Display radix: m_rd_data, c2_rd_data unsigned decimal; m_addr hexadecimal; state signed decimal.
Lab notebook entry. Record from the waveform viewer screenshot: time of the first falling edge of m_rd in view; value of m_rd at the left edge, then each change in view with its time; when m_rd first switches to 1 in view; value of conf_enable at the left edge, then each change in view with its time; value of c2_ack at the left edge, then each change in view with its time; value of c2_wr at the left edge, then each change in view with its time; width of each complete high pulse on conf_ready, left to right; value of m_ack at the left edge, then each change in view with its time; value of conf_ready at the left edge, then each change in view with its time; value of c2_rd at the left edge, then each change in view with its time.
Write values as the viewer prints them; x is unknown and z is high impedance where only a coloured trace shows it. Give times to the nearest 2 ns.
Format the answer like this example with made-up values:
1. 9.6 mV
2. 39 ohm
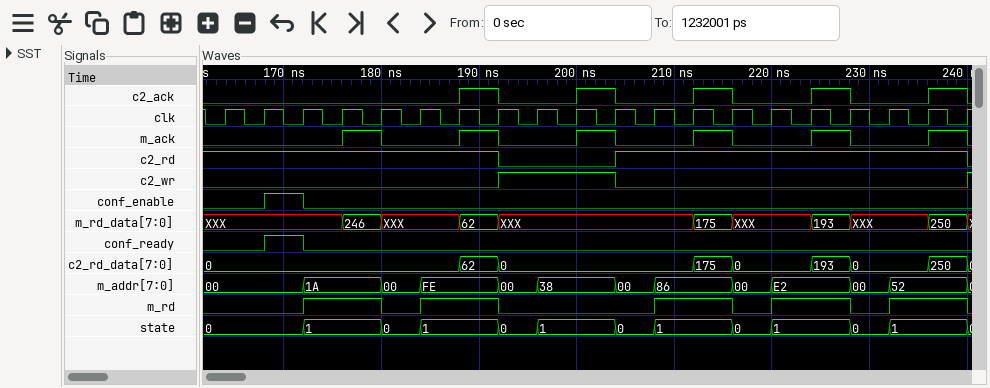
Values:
1. 180 ns
2. 0, 1 at 172 ns, 0 at 180 ns, 1 at 184 ns, 0 at 192 ns, 1 at 208 ns, 0 at 216 ns, 1 at 220 ns, 0 at 228 ns, 1 at 232 ns, 0 at 240 ns
3. 172 ns
4. 0, 1 at 168 ns, 0 at 172 ns
5. 0, 1 at 188 ns, 0 at 192 ns, 1 at 200 ns, 0 at 204 ns, 1 at 212 ns, 0 at 216 ns, 1 at 224 ns, 0 at 228 ns, 1 at 236 ns, 0 at 240 ns
6. 0, 1 at 192 ns, 0 at 204 ns, 1 at 240 ns
7. 4 ns
8. 0, 1 at 176 ns, 0 at 180 ns, 1 at 188 ns, 0 at 192 ns, 1 at 200 ns, 0 at 204 ns, 1 at 212 ns, 0 at 216 ns, 1 at 224 ns, 0 at 228 ns, 1 at 236 ns, 0 at 240 ns
9. 0, 1 at 168 ns, 0 at 172 ns
10. 1, 0 at 192 ns, 1 at 204 ns, 0 at 240 ns
